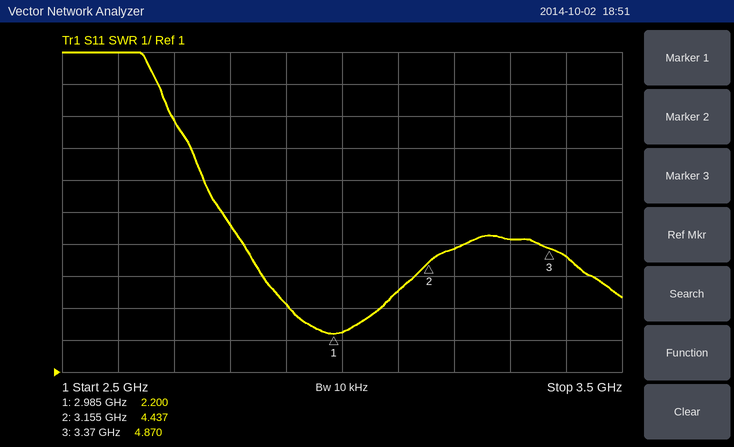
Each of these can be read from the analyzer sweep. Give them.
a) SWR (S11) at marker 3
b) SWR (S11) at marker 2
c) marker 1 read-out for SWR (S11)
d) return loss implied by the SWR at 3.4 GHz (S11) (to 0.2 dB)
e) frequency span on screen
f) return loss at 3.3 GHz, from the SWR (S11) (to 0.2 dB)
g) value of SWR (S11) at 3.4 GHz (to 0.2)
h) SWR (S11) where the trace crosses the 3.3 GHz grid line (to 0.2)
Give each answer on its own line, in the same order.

4.870
4.437
2.200
3.8 dB
1 GHz
3.4 dB
4.6
5.2
